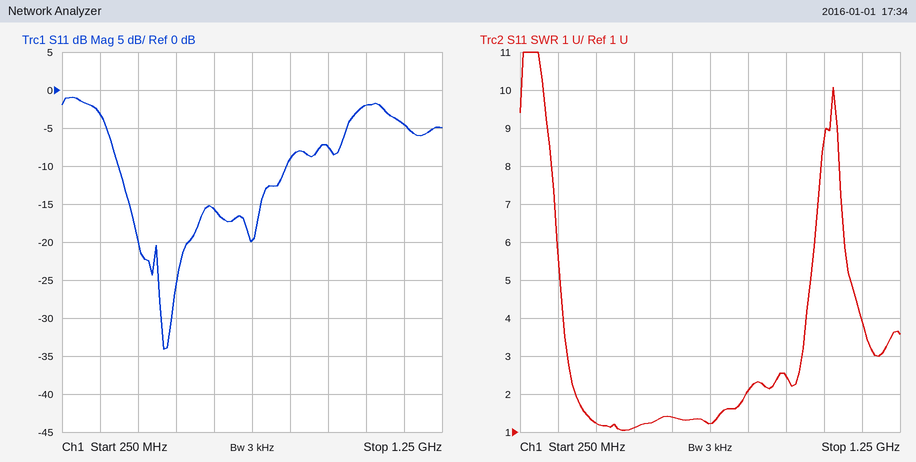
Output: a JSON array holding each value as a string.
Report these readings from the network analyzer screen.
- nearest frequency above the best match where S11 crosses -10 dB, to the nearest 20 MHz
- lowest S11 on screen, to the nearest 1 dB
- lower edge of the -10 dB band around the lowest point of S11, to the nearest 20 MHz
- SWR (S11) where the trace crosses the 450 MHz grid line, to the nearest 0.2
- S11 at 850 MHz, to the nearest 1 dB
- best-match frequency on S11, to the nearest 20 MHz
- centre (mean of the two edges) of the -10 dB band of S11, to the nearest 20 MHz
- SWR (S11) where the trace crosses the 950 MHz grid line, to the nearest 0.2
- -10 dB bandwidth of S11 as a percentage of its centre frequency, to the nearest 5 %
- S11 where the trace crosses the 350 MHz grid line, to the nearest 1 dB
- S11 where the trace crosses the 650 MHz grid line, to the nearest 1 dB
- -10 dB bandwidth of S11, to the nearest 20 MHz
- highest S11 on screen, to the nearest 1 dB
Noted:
["840 MHz", "-34 dB", "400 MHz", "1.2", "-9 dB", "520 MHz", "620 MHz", "2.4", "70 %", "-3 dB", "-16 dB", "440 MHz", "-1 dB"]
